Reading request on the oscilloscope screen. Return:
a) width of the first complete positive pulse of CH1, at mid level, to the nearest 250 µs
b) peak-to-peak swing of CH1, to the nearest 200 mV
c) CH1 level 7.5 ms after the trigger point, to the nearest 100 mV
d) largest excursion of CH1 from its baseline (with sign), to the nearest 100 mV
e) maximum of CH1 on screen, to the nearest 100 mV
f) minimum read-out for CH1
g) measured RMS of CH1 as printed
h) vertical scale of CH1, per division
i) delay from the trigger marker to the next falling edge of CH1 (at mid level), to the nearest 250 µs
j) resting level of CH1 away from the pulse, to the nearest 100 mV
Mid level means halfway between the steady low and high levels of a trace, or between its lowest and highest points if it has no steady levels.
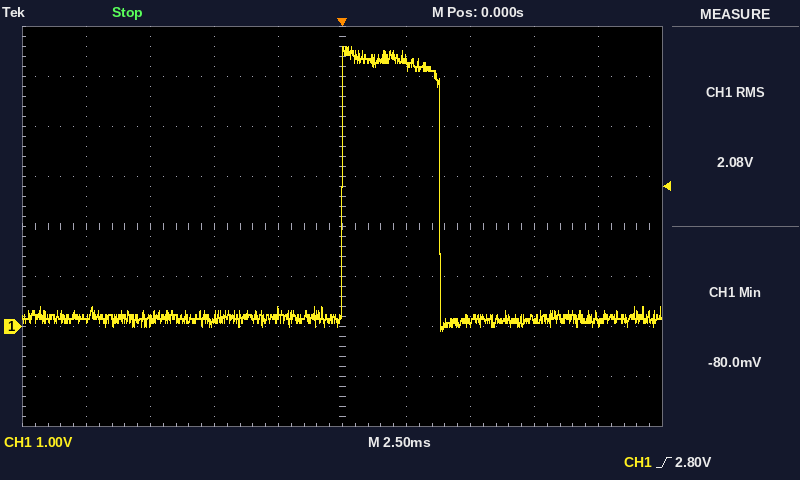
3.75 ms
5.6 V
200 mV
+5.4 V
5.6 V
-80.0 mV
2.08 V
1 V
3.75 ms
200 mV
